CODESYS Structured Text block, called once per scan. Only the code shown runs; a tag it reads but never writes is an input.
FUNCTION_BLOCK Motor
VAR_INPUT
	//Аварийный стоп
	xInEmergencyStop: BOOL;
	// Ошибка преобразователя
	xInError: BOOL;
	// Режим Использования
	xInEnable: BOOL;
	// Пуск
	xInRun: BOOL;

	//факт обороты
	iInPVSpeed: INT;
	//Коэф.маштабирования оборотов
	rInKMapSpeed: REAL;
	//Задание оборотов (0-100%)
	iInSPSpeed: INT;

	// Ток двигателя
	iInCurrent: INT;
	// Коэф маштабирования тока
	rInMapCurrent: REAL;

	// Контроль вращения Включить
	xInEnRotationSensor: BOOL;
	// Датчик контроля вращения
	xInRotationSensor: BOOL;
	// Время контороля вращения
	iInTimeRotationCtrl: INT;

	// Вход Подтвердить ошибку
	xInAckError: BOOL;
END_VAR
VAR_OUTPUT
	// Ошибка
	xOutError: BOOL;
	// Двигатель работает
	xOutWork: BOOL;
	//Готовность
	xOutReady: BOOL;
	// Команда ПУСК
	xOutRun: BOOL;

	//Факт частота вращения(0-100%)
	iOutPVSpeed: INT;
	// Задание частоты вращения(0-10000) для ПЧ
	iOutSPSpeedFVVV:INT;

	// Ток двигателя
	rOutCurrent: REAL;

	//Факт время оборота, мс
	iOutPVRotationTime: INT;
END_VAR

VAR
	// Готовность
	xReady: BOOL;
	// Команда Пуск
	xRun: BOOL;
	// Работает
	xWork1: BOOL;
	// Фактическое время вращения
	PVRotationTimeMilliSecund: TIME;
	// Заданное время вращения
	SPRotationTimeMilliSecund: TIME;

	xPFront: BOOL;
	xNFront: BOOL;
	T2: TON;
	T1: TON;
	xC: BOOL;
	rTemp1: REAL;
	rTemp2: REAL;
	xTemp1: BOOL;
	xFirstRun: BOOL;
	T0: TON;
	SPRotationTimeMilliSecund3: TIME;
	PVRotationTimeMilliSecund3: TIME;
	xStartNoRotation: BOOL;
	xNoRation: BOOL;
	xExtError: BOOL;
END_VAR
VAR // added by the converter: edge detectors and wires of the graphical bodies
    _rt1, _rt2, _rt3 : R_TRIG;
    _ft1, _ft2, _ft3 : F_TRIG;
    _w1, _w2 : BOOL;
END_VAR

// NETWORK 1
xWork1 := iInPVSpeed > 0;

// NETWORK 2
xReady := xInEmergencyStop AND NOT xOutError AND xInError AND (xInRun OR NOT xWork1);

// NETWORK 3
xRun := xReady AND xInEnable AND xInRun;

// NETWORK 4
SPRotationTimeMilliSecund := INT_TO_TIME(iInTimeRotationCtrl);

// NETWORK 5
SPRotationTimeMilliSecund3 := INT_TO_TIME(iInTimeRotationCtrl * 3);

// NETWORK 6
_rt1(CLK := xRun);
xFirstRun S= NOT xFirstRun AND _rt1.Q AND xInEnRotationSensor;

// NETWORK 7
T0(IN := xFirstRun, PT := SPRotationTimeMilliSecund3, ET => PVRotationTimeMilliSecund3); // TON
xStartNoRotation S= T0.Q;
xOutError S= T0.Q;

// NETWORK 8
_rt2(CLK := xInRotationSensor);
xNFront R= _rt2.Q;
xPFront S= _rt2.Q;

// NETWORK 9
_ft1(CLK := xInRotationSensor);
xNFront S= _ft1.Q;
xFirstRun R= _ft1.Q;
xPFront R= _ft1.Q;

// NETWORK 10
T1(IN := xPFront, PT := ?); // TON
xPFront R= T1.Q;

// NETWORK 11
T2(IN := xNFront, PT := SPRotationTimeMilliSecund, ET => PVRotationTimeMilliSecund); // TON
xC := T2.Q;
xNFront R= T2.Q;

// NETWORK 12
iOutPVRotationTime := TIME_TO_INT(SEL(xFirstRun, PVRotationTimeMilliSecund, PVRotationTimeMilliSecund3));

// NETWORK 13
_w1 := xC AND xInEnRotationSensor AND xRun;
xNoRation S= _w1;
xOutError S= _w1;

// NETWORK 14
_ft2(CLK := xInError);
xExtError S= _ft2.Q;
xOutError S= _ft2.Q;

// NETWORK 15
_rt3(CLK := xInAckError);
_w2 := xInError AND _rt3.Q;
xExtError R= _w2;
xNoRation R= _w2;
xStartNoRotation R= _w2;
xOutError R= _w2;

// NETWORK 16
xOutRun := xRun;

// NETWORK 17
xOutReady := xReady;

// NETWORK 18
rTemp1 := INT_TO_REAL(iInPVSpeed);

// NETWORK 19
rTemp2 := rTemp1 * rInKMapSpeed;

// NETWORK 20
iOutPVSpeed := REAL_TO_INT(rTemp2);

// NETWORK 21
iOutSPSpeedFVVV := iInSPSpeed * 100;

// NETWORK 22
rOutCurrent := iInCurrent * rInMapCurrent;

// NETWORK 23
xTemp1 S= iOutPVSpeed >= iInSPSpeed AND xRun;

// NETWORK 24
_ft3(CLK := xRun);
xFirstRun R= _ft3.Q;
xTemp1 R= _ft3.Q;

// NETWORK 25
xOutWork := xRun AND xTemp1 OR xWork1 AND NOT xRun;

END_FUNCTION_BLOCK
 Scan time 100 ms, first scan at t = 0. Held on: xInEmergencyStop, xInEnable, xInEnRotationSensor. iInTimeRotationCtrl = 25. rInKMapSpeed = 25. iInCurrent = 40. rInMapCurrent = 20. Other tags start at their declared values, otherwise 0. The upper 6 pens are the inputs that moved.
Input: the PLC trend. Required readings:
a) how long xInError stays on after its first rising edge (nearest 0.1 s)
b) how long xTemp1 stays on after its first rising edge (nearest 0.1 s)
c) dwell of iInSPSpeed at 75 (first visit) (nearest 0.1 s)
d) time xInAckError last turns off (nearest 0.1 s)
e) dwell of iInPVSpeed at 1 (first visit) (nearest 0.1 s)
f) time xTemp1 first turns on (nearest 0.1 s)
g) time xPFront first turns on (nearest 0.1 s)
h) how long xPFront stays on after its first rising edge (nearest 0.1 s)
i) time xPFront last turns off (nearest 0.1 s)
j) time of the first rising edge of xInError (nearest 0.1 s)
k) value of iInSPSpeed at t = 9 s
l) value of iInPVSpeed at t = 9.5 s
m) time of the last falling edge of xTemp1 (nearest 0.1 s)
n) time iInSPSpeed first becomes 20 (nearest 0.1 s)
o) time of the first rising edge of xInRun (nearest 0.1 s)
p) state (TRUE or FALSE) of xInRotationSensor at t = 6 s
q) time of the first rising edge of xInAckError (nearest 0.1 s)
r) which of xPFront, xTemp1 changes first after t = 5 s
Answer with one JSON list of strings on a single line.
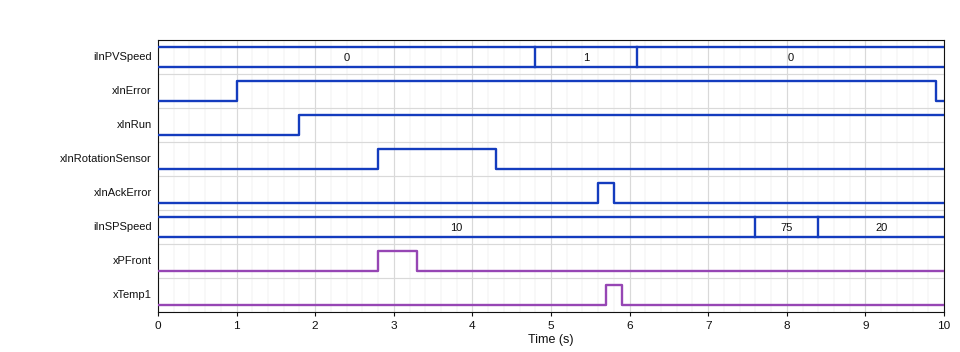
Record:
["8.9 s", "0.2 s", "0.8 s", "5.8 s", "1.3 s", "5.7 s", "2.8 s", "0.5 s", "3.3 s", "1.0 s", "20", "0", "5.9 s", "8.4 s", "1.8 s", "FALSE", "5.6 s", "xTemp1"]
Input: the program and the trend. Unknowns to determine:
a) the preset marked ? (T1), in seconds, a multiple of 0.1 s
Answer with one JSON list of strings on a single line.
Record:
["0.5 s"]
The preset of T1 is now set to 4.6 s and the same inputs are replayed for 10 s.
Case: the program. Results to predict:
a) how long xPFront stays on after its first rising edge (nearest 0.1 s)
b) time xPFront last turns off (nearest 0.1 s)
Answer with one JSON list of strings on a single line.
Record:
["1.5 s", "4.3 s"]
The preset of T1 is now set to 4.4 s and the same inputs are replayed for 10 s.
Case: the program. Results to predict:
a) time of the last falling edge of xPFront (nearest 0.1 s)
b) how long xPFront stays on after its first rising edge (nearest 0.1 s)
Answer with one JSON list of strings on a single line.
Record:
["4.3 s", "1.5 s"]
